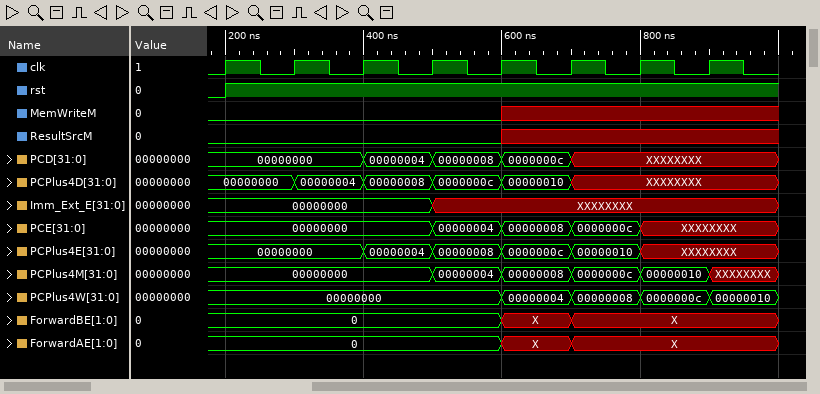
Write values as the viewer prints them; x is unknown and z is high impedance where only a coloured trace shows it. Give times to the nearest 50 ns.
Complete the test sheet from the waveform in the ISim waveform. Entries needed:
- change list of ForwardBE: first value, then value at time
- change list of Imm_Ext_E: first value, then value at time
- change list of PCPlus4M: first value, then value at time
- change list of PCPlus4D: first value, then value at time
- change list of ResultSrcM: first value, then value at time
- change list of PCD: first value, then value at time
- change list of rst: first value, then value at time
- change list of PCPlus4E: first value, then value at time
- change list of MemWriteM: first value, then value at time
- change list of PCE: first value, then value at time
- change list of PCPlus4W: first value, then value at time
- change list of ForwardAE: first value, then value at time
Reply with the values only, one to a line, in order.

0, X at 600 ns, X at 700 ns
00000000, XXXXXXXX at 500 ns
00000000, 00000004 at 500 ns, 00000008 at 600 ns, 0000000c at 700 ns, 00000010 at 800 ns, XXXXXXXX at 900 ns
00000000, 00000004 at 300 ns, 00000008 at 400 ns, 0000000c at 500 ns, 00000010 at 600 ns, XXXXXXXX at 700 ns
0, x at 600 ns
00000000, 00000004 at 400 ns, 00000008 at 500 ns, 0000000c at 600 ns, XXXXXXXX at 700 ns
0, 1 at 200 ns
00000000, 00000004 at 400 ns, 00000008 at 500 ns, 0000000c at 600 ns, 00000010 at 700 ns, XXXXXXXX at 800 ns
0, x at 600 ns
00000000, 00000004 at 500 ns, 00000008 at 600 ns, 0000000c at 700 ns, XXXXXXXX at 800 ns
00000000, 00000004 at 600 ns, 00000008 at 700 ns, 0000000c at 800 ns, 00000010 at 900 ns
0, X at 600 ns, X at 700 ns
